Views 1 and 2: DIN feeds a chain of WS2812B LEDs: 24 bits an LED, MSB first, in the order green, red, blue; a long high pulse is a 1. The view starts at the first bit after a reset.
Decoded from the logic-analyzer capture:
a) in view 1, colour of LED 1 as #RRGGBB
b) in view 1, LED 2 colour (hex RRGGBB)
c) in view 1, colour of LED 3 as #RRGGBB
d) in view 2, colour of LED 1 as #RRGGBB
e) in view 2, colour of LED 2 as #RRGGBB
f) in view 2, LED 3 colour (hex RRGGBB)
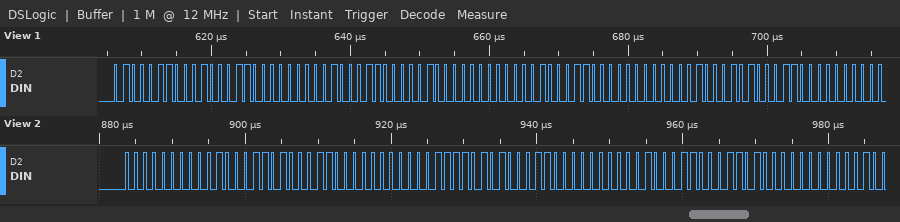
#234600
#084600
#004611
#230046
#3D0046
#460034
